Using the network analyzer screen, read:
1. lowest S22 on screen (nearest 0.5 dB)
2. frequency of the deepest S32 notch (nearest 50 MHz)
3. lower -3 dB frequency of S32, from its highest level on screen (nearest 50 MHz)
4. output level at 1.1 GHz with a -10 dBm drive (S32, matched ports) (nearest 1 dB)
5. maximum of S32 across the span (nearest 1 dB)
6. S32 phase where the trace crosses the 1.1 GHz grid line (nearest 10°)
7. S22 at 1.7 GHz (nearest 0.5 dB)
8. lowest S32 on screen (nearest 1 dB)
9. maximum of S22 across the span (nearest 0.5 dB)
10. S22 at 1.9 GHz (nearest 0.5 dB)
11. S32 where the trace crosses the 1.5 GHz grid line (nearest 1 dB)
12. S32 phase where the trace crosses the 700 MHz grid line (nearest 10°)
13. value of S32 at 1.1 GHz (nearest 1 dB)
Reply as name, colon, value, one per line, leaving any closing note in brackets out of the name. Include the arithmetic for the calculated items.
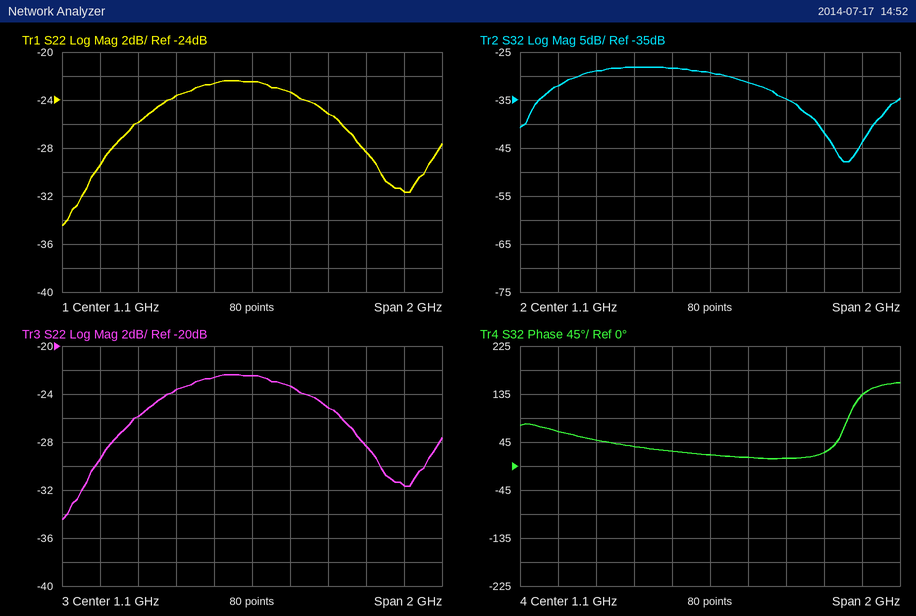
lowest S22 on screen: -34.5 dB
frequency of the deepest S32 notch: 1.80 GHz
lower -3 dB frequency of S32, from its highest level on screen: 350 MHz
output level at 1.1 GHz with a -10 dBm drive (S32, matched ports): -10 dBm + (-29 dB) = -39 dBm
maximum of S32 across the span: -28 dB
S32 phase where the trace crosses the 1.1 GHz grid line: 20°
S22 at 1.7 GHz: -28.5 dB
lowest S32 on screen: -48 dB
maximum of S22 across the span: -22.5 dB
S22 at 1.9 GHz: -31.5 dB
S32 where the trace crosses the 1.5 GHz grid line: -35 dB
S32 phase where the trace crosses the 700 MHz grid line: 40°
value of S32 at 1.1 GHz: -29 dB
